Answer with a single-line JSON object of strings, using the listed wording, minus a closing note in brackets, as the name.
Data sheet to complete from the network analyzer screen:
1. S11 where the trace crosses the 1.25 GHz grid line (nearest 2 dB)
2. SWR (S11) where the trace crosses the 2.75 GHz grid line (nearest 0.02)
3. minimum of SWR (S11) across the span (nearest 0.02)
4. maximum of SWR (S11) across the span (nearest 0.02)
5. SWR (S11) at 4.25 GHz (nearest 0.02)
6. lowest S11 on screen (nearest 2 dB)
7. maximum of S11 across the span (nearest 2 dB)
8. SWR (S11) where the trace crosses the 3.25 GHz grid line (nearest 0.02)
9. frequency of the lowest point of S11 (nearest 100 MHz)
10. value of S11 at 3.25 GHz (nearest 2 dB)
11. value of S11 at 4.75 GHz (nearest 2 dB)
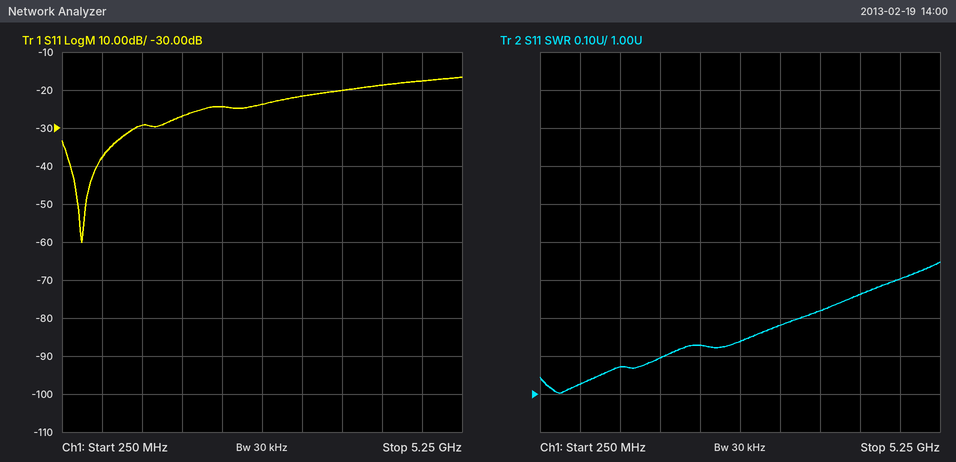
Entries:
{"S11 where the trace crosses the 1.25 GHz grid line": "-30 dB", "SWR (S11) where the trace crosses the 2.75 GHz grid line": "1.14", "minimum of SWR (S11) across the span": "1.00", "maximum of SWR (S11) across the span": "1.34", "SWR (S11) at 4.25 GHz": "1.26", "lowest S11 on screen": "-60 dB", "maximum of S11 across the span": "-16 dB", "SWR (S11) where the trace crosses the 3.25 GHz grid line": "1.18", "frequency of the lowest point of S11": "500 MHz", "value of S11 at 3.25 GHz": "-22 dB", "value of S11 at 4.75 GHz": "-18 dB"}
